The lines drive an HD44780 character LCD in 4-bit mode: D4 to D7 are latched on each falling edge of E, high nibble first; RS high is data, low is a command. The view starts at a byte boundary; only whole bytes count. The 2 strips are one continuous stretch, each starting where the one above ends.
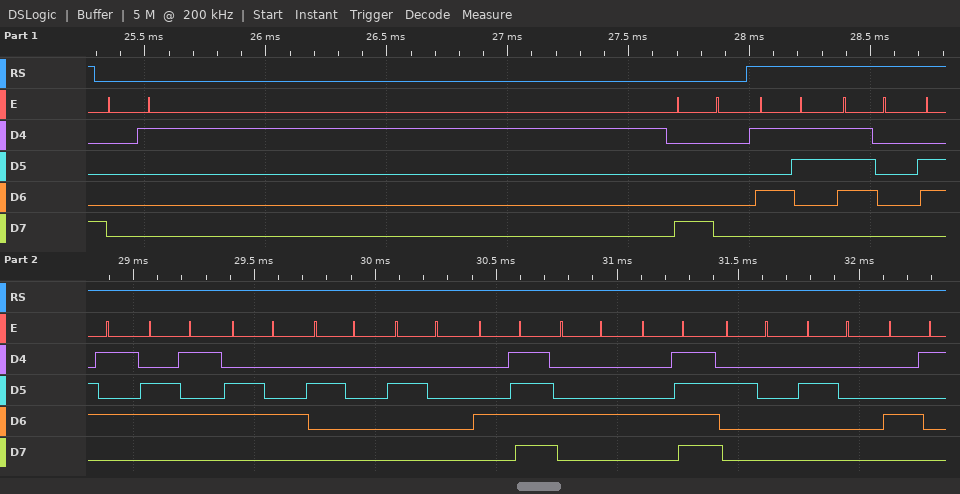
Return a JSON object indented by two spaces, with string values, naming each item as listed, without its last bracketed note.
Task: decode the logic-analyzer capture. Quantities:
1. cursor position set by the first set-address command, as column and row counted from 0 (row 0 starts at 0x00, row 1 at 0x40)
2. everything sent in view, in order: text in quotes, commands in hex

{
  "cursor position set by the first set-address command, as column and row counted from 0": "column 0, row 0",
  "everything sent in view, in order: text in quotes, commands in hex": "0x01 0x80 \"Speed  ODO  A\""
}
